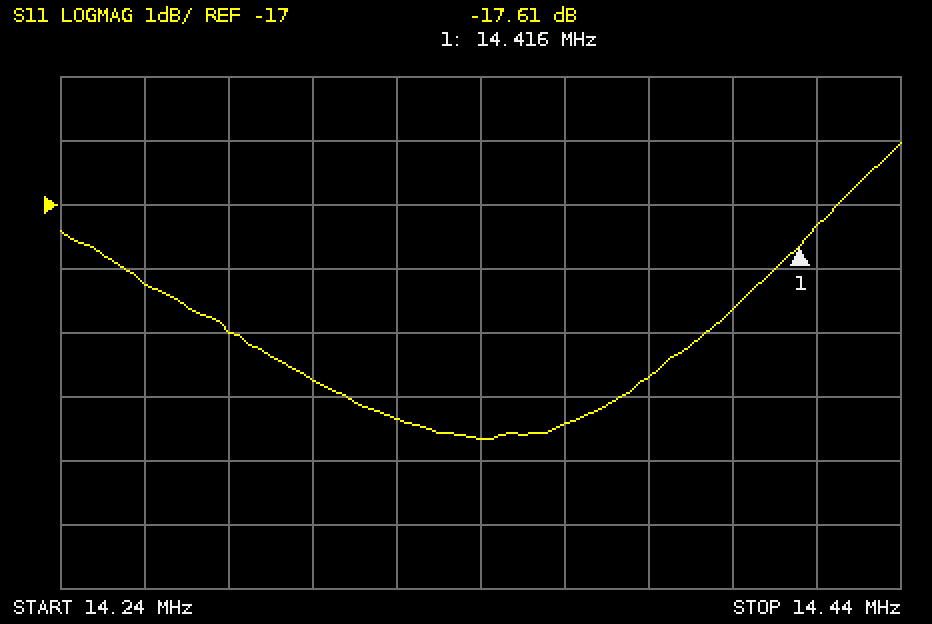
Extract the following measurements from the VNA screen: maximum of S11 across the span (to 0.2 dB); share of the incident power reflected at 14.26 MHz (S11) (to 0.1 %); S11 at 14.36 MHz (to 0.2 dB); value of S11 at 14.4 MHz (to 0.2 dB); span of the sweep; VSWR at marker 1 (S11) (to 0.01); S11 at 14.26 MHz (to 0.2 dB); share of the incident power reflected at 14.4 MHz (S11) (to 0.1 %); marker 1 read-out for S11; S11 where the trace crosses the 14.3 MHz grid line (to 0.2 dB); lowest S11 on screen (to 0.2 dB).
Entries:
-16.0 dB
1.5 %
-20.4 dB
-18.6 dB
200 kHz
1.30
-18.2 dB
1.4 %
-17.61 dB
-19.8 dB
-20.6 dB
